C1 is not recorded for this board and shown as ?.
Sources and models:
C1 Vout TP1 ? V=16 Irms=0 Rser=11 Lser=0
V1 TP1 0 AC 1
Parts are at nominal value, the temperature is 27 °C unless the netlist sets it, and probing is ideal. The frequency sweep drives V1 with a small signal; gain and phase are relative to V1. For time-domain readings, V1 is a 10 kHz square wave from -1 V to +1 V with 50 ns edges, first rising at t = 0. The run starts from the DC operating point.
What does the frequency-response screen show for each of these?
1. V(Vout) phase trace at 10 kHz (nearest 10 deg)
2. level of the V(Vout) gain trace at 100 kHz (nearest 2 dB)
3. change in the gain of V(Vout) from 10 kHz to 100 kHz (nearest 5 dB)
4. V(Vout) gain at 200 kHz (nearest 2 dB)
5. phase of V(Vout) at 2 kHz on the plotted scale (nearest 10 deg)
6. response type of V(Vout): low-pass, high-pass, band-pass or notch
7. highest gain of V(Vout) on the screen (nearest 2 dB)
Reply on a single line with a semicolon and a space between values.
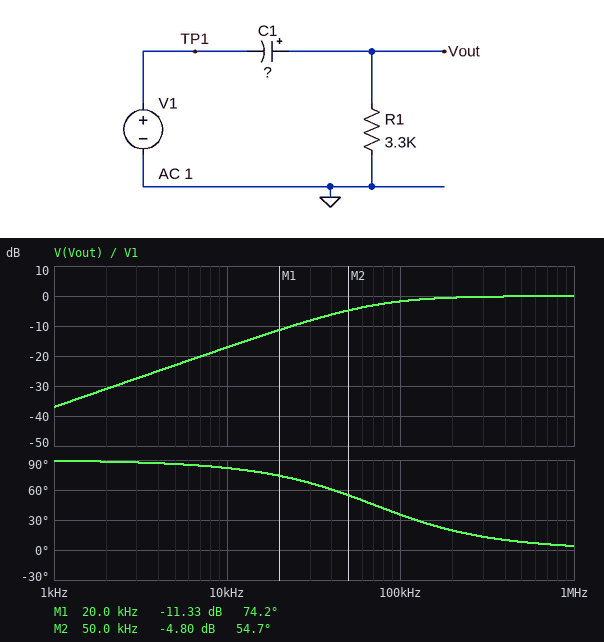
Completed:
80 deg; -2 dB; 15 dB; 0 dB; 90 deg; high-pass; 0 dB
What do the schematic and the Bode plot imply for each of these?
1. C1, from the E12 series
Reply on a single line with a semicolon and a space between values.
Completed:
680 pF
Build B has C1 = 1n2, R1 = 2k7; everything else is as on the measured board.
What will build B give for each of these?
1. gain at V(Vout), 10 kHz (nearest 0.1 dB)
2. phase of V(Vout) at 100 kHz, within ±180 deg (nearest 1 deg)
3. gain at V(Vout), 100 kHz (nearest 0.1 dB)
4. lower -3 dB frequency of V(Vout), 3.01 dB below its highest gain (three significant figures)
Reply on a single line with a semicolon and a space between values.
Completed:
-14.0 dB; 26 deg; -1.0 dB; 48.9 kHz
